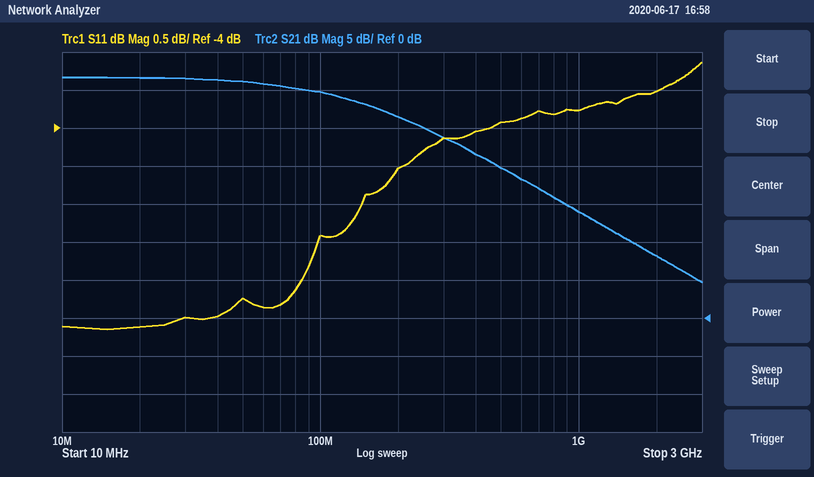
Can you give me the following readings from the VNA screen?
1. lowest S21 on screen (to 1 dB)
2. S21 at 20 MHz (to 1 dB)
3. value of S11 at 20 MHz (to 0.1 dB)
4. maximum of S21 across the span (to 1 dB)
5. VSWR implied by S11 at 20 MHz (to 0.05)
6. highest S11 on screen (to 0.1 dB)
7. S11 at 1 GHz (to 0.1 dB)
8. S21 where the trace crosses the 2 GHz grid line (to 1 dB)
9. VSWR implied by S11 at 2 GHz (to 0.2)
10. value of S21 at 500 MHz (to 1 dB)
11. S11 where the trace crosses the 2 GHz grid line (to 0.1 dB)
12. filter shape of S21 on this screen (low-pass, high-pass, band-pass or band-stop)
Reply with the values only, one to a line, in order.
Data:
5 dB
32 dB
-6.6 dB
32 dB
2.75
-3.1 dB
-3.8 dB
8 dB
5.0
20 dB
-3.5 dB
low-pass
